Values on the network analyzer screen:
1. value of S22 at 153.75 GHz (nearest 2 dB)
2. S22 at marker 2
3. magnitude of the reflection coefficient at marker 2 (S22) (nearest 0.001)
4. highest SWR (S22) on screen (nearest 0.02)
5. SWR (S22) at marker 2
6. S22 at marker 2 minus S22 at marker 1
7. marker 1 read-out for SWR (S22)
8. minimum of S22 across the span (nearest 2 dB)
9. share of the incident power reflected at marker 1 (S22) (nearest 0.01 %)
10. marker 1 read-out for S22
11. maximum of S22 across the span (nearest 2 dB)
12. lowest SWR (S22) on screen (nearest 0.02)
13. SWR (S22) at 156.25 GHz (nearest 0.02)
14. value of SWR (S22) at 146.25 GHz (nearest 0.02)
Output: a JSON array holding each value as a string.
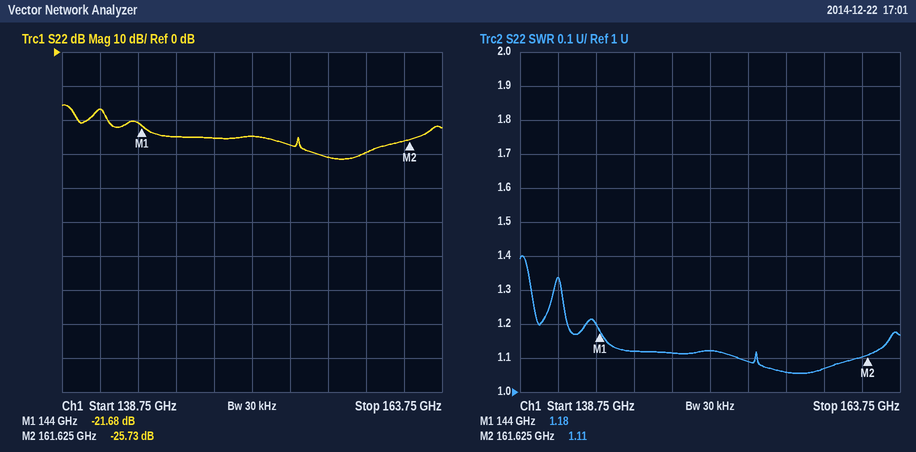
["-28 dB", "-25.73 dB", "0.052", "1.40", "1.11", "-4.05 dB", "1.18", "-32 dB", "0.68 %", "-21.68 dB", "-16 dB", "1.06", "1.06", "1.12"]
